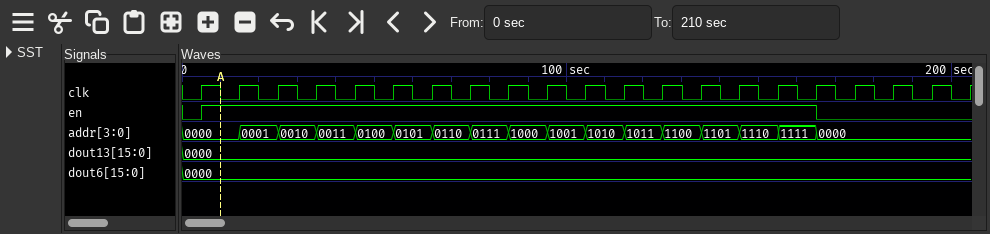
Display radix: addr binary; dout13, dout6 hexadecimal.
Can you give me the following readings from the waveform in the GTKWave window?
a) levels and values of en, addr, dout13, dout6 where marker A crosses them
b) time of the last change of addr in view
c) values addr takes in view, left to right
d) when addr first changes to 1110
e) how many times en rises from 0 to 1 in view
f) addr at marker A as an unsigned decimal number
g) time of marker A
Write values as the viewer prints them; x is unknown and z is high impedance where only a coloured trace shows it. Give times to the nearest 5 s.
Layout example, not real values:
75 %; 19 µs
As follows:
en=1, addr=0000, dout13=0000, dout6=0000; 165 s; 0000, 0001, 0010, 0011, 0100, 0101, 0110, 0111, 1000, 1001, 1010, 1011, 1100, 1101, 1110, 1111, 0000; 145 s; 1; 0; 10 s
